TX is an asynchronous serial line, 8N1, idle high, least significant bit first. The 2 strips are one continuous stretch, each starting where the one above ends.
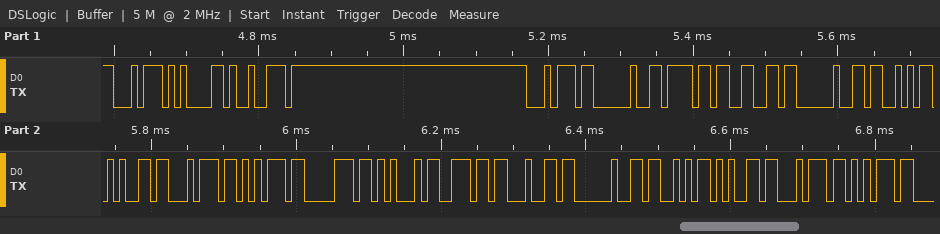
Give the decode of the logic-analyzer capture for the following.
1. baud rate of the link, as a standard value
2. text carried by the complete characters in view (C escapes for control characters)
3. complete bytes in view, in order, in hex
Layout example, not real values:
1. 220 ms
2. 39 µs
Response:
1. 115200 baud
2. "tart of SetupEnd Setu"
3. 74 61 72 74 20 6F 66 20 53 65 74 75 70 45 6E 64 20 53 65 74 75
